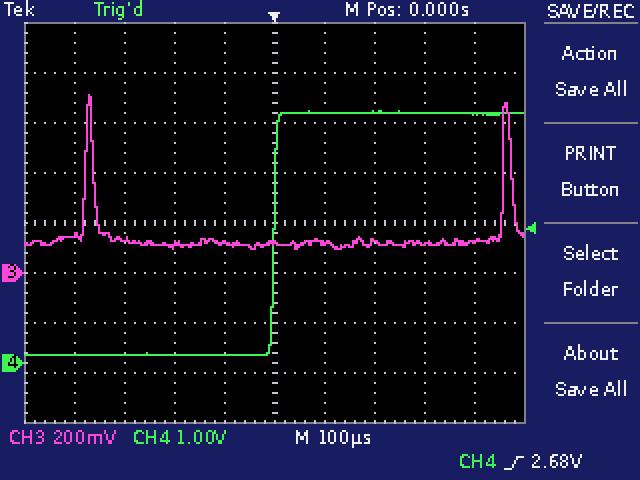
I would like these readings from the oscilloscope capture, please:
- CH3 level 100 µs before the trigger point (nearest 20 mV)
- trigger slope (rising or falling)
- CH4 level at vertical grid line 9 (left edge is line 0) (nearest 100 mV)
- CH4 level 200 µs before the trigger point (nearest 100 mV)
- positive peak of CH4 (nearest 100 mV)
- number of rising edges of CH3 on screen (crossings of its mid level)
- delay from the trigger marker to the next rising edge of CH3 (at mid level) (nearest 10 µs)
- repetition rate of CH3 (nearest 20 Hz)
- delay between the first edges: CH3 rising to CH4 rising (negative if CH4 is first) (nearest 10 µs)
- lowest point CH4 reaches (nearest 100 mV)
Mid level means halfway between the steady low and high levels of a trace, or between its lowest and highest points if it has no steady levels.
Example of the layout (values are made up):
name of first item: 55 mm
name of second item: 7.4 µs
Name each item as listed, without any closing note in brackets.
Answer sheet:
CH3 level 100 µs before the trigger point: 120 mV
trigger slope: rising
CH4 level at vertical grid line 9 (left edge is line 0): 5.0 V
CH4 level 200 µs before the trigger point: 200 mV
positive peak of CH4: 5.0 V
number of rising edges of CH3 on screen: 2
delay from the trigger marker to the next rising edge of CH3 (at mid level): 460 µs
repetition rate of CH3: 1.20 kHz
delay between the first edges: CH3 rising to CH4 rising (negative if CH4 is first): +380 µs
lowest point CH4 reaches: 200 mV
